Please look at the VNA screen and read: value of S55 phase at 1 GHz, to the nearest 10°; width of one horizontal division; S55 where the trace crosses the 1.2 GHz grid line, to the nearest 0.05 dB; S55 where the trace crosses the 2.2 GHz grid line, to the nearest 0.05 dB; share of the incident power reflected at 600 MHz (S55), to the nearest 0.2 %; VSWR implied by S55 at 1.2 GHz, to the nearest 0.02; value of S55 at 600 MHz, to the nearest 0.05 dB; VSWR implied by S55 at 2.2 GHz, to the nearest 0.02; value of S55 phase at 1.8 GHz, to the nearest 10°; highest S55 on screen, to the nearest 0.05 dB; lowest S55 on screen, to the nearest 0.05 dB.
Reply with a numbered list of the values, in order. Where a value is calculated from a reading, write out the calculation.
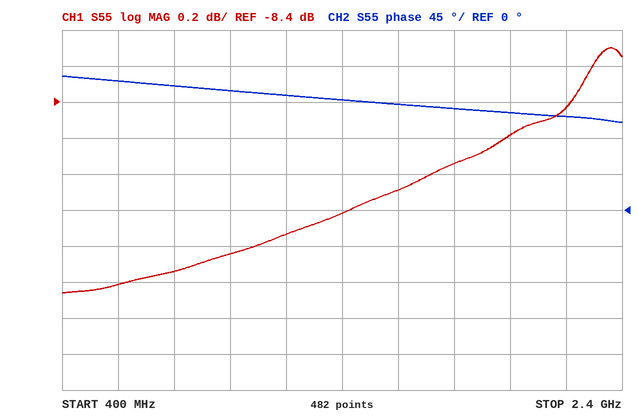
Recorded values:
1. 150°
2. 200 MHz
3. -9.15 dB
4. -8.45 dB
5. 10^(-9.4/10) ≈ 11.5 %, so 11.4 % to the nearest 0.2 %
6. |Γ| = 10^(-9.15/20) = 0.3487; VSWR = (1 + 0.3487)/(1 − 0.3487) ≈ 2.07, so 2.08 to the nearest 0.02
7. -9.40 dB
8. |Γ| = 10^(-8.45/20) = 0.3780; VSWR = (1 + 0.3780)/(1 − 0.3780) ≈ 2.22
9. 130°
10. -8.10 dB
11. -9.45 dB
